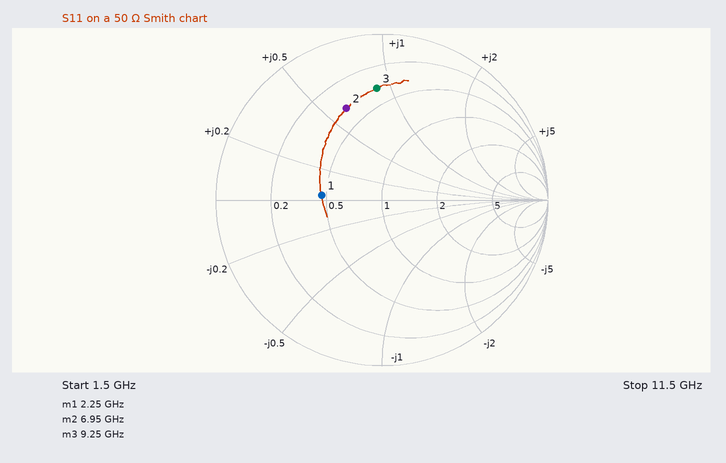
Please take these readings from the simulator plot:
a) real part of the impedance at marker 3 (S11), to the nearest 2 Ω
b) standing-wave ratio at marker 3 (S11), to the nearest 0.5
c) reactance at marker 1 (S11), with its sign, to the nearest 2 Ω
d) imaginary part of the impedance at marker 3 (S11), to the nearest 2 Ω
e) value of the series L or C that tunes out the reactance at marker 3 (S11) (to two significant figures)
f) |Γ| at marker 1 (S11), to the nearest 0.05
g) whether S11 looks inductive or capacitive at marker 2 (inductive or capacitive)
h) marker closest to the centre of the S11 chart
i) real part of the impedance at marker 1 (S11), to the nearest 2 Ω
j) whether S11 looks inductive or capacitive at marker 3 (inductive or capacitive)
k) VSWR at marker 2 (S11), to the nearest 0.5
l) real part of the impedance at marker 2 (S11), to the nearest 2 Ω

18 Ω
5.0
+2 Ω
+44 Ω
390 fF
0.35
inductive
marker 1
24 Ω
inductive
4.0
18 Ω
